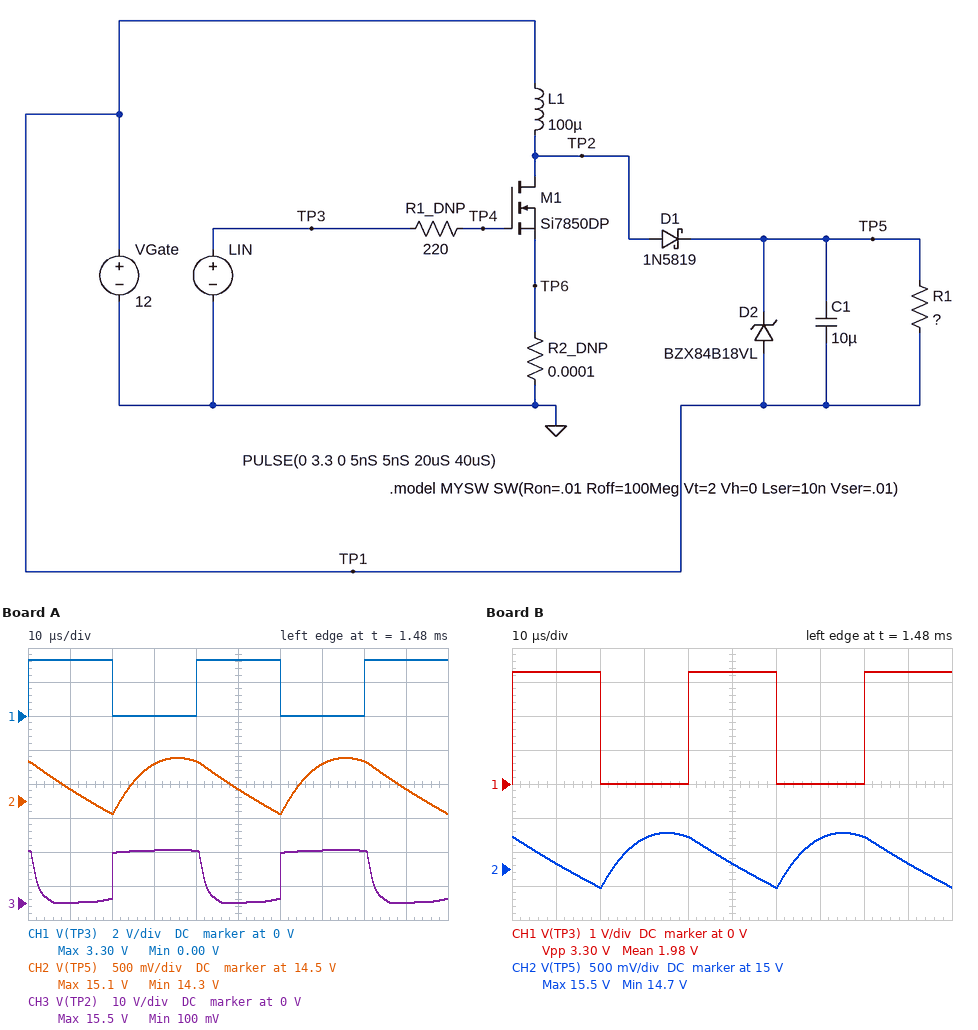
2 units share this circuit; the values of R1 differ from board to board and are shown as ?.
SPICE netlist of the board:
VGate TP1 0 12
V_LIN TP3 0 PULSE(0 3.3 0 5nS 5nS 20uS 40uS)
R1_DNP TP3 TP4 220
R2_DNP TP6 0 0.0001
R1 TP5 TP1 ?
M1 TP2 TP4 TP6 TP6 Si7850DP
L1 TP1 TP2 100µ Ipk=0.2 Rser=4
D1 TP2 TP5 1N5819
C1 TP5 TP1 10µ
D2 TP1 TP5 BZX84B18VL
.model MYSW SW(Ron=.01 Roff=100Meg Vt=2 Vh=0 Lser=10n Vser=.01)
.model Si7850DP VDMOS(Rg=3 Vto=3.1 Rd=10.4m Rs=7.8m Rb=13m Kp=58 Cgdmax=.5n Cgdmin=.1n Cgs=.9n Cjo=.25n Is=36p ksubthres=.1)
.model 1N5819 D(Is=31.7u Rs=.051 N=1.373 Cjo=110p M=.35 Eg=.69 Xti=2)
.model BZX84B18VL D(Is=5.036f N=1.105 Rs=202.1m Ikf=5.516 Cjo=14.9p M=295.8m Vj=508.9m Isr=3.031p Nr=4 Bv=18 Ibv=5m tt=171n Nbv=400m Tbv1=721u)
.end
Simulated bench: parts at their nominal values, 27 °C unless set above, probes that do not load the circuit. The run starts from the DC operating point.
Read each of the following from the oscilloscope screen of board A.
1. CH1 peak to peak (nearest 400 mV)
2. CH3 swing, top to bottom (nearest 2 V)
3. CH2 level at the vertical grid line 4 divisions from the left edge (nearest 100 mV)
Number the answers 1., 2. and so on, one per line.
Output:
1. 3.2 V
2. 16 V
3. 15.1 V
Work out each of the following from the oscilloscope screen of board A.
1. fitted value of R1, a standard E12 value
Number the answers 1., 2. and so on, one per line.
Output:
1. 6.8 Ω
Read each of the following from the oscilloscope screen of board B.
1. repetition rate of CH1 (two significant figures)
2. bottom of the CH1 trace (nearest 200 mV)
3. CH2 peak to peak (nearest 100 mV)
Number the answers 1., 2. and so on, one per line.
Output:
1. 25 kHz
2. 0 V
3. 800 mV
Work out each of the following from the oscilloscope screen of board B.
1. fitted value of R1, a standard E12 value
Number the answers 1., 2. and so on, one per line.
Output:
1. 8.2 Ω
